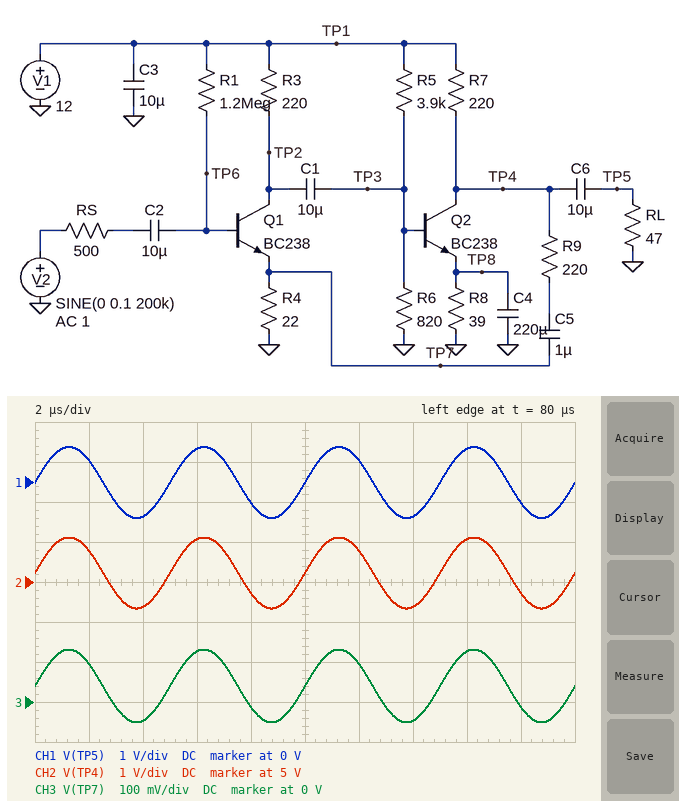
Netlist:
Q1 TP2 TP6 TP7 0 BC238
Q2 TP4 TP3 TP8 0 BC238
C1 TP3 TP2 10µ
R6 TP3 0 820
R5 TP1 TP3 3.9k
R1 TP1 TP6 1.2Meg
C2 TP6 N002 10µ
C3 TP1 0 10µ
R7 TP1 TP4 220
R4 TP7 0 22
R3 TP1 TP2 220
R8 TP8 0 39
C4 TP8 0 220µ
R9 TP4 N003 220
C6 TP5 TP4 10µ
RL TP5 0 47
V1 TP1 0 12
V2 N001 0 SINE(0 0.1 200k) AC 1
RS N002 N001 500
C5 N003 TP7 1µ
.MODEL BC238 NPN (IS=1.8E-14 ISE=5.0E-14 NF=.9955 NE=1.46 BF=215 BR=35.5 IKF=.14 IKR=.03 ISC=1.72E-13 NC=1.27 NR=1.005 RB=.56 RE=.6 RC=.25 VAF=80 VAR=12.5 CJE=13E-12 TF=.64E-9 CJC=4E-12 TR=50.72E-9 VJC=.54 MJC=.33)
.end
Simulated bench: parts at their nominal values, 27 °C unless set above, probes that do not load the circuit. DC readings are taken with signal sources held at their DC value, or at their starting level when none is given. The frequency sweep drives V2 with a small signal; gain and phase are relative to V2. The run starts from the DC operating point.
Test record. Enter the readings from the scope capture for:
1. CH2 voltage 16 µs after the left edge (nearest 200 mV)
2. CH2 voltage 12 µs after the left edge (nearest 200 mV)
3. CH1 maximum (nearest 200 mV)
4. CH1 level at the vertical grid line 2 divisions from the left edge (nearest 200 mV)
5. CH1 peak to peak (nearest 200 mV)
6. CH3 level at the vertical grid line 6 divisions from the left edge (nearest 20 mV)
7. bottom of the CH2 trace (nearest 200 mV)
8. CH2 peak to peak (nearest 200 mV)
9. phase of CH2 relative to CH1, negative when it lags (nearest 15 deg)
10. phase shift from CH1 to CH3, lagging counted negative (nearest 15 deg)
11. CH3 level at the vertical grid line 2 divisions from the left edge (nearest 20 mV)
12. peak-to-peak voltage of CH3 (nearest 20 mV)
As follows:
6.0 V
5.8 V
800 mV
-800 mV
1.8 V
100 mV
4.4 V
1.8 V
0 deg
0 deg
-40 mV
180 mV
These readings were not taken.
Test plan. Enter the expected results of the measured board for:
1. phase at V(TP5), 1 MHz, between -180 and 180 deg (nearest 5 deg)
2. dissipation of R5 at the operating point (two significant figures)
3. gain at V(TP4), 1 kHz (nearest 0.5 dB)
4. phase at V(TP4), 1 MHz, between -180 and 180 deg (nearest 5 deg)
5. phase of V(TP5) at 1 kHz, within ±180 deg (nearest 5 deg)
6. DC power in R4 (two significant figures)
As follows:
-5 deg
26 mW
20.5 dB
-5 deg
-10 deg
74 µW
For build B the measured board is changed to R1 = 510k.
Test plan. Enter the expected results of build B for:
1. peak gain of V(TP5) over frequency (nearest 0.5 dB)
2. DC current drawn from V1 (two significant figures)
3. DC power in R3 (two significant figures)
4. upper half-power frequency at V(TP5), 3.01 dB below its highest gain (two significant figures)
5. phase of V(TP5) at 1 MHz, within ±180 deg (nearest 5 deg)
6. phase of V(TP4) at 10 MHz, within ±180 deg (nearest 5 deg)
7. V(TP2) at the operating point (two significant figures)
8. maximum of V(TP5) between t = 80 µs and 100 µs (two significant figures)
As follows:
24.5 dB
38 mA
4.1 mW
600 Hz
-5 deg
-40 deg
11 V
900 mV
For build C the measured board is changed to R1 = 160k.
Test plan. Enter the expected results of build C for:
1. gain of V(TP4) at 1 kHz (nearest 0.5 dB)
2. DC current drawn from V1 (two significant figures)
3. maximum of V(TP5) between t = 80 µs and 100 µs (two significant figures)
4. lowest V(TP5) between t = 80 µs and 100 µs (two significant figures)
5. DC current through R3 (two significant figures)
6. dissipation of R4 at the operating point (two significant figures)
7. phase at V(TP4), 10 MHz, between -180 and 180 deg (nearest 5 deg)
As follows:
21.0 dB
46 mA
910 mV
-960 mV
13 mA
3.7 mW
-40 deg
